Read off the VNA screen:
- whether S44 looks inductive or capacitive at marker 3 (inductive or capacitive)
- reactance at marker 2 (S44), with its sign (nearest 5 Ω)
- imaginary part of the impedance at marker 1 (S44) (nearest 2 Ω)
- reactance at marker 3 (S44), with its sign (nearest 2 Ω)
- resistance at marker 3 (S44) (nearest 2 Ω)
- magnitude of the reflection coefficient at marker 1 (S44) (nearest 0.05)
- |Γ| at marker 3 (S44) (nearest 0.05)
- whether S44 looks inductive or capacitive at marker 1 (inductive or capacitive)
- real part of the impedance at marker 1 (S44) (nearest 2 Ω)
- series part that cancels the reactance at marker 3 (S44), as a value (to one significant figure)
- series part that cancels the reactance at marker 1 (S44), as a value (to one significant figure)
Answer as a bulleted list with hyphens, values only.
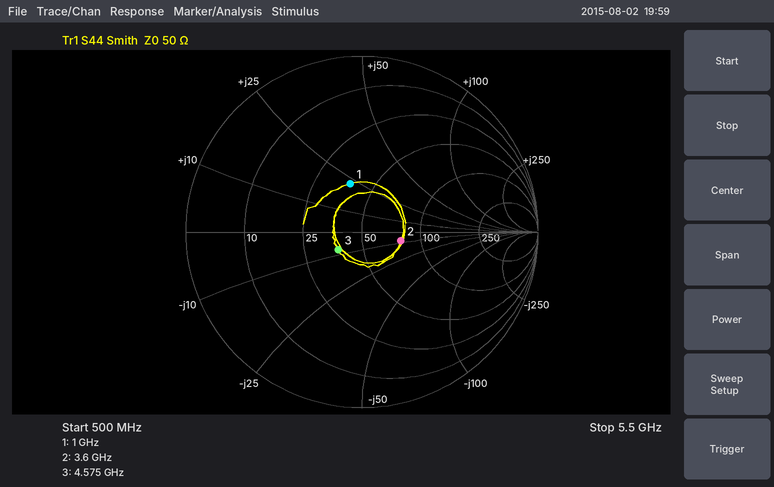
- capacitive
- -10 Ω
- +22 Ω
- -8 Ω
- 38 Ω
- 0.30
- 0.15
- inductive
- 38 Ω
- 300 pH
- 7 pF
